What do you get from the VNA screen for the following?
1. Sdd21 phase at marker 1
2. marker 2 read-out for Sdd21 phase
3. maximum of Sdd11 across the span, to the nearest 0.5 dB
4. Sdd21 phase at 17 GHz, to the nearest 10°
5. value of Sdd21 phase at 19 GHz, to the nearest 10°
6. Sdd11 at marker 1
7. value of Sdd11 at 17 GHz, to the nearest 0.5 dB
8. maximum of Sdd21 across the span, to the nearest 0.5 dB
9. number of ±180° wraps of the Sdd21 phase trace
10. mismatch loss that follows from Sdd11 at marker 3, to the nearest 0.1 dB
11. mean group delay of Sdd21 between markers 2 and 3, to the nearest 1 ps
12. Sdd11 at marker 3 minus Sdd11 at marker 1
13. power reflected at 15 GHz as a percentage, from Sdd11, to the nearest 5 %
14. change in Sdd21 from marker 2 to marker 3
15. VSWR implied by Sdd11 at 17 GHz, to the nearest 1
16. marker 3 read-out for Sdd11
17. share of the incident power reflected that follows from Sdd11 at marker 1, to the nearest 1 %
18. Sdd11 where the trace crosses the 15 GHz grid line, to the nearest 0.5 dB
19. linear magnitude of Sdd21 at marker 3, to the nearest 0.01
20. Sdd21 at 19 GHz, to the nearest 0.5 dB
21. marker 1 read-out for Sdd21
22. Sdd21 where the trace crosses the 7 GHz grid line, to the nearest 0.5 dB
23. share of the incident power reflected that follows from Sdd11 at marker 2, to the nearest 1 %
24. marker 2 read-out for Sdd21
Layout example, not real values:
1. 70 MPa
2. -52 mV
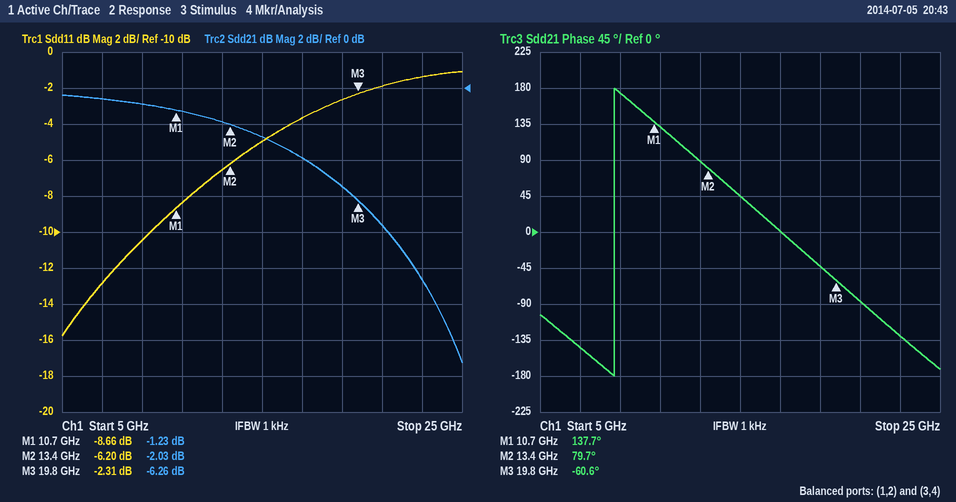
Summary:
1. 137.7°
2. 79.7°
3. -1.0 dB
4. 0°
5. -40°
6. -8.66 dB
7. -3.5 dB
8. -0.5 dB
9. 1
10. 3.8 dB
11. 61 ps
12. 6.35 dB
13. 30 %
14. -4.23 dB
15. 5
16. -2.31 dB
17. 14 %
18. -5.0 dB
19. 0.49
20. -5.5 dB
21. -1.23 dB
22. -0.5 dB
23. 24 %
24. -2.03 dB
